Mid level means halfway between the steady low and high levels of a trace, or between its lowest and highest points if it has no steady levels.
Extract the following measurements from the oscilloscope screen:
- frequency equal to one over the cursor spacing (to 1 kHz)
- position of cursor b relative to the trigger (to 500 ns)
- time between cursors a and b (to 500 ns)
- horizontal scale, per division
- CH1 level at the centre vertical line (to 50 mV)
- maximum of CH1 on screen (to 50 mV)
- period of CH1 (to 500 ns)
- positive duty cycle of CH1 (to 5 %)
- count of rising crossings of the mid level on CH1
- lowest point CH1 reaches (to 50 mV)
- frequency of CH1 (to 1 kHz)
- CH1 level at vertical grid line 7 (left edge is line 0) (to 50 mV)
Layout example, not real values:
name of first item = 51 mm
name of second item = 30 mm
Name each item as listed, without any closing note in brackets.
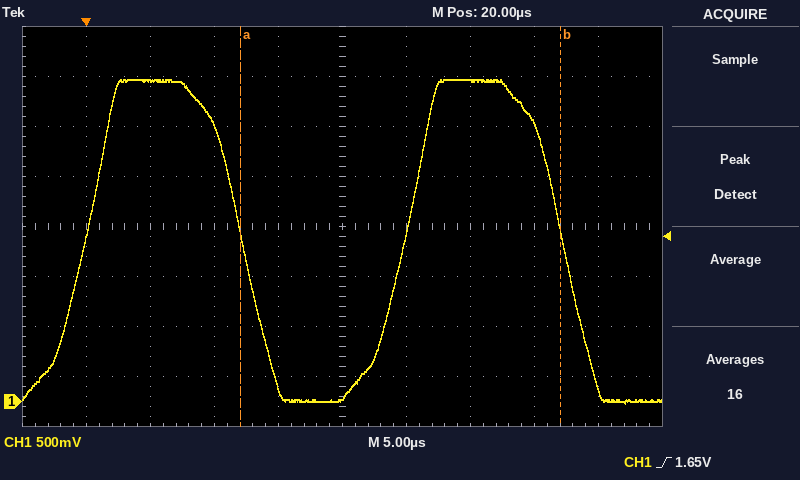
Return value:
frequency equal to one over the cursor spacing = 40 kHz
position of cursor b relative to the trigger = +37.0 µs
time between cursors a and b = 25.0 µs
horizontal scale, per division = 5 µs
CH1 level at the centre vertical line = 50 mV
maximum of CH1 on screen = 3.20 V
period of CH1 = 25.0 µs
positive duty cycle of CH1 = 50 %
count of rising crossings of the mid level on CH1 = 2
lowest point CH1 reaches = 0 mV
frequency of CH1 = 40 kHz
CH1 level at vertical grid line 7 (left edge is line 0) = 3.20 V
